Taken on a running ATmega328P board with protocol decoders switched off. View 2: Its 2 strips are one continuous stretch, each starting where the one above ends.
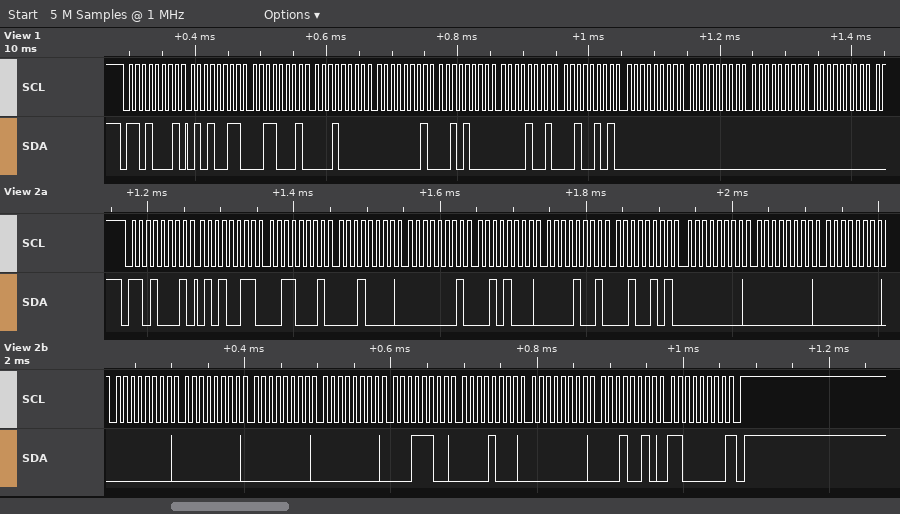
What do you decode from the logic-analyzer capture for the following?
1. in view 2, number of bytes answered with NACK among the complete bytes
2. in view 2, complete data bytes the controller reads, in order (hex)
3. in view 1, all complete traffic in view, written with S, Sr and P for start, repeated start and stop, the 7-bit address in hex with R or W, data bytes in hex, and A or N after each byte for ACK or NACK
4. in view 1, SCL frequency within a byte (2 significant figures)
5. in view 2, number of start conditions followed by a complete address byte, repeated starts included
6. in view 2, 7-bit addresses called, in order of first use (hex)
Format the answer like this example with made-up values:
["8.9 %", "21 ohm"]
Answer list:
["1", "53 31 10 01 28 09 25 00 00 00 00 00 00 00 1C 08 00 12 C0", "S 68R A 53 A 31 A 10 A 01 A 28 A 09 A 25 A 00 A 00 A 00 A 00 A", "100 kHz", "1", "0x68"]
